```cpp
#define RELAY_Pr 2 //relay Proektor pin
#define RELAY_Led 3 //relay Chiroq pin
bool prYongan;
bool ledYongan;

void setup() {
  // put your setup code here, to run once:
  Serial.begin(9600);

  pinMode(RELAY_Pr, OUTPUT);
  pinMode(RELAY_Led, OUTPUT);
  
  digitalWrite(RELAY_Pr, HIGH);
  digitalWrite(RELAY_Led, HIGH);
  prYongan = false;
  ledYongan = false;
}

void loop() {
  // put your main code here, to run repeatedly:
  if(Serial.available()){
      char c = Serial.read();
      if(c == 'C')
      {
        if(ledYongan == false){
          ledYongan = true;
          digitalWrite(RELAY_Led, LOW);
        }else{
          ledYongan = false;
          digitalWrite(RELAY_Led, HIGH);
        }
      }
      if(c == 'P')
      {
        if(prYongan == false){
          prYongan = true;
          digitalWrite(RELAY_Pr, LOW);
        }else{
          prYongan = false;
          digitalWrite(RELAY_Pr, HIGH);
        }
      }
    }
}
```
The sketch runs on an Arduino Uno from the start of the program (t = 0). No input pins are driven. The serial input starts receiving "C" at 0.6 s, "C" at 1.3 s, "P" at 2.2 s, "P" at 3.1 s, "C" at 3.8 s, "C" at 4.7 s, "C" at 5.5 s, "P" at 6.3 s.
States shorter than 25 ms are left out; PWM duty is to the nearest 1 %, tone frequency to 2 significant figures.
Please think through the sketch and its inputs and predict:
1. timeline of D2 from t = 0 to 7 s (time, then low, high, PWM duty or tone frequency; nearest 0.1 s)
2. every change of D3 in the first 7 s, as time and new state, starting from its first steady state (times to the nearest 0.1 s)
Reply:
0 s high; 2.2 s low; 3.1 s high; 6.3 s low
0 s high; 0.6 s low; 1.3 s high; 3.8 s low; 4.7 s high; 5.5 s low
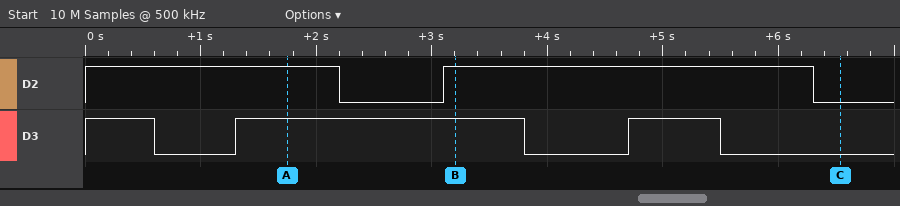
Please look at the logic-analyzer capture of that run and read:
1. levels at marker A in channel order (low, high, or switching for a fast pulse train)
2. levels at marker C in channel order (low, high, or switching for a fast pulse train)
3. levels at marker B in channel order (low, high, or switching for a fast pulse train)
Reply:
D2 high, D3 high
D2 low, D3 low
D2 high, D3 high
